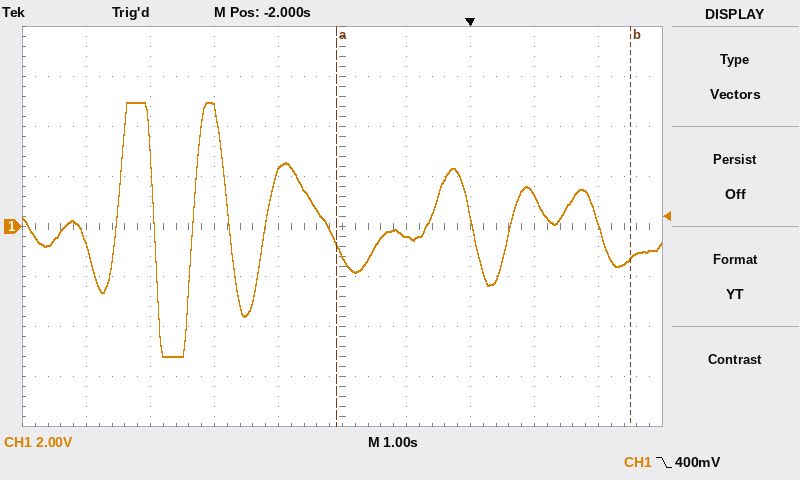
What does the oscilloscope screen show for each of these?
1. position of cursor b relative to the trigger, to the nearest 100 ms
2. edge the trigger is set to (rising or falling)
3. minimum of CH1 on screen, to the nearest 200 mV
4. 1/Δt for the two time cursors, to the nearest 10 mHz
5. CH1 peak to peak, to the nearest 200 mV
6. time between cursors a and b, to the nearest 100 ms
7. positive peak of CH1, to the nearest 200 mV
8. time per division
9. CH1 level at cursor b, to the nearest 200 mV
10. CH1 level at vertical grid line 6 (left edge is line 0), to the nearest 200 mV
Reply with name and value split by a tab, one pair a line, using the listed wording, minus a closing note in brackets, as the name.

position of cursor b relative to the trigger, to the nearest 100 ms	+2.5 s
edge the trigger is set to	falling
minimum of CH1 on screen, to the nearest 200 mV	-5.2 V
1/Δt for the two time cursors, to the nearest 10 mHz	220 mHz
CH1 peak to peak, to the nearest 200 mV	10.2 V
time between cursors a and b, to the nearest 100 ms	4.6 s
positive peak of CH1, to the nearest 200 mV	5.0 V
time per division	1 s
CH1 level at cursor b, to the nearest 200 mV	-1.2 V
CH1 level at vertical grid line 6 (left edge is line 0), to the nearest 200 mV	-400 mV
